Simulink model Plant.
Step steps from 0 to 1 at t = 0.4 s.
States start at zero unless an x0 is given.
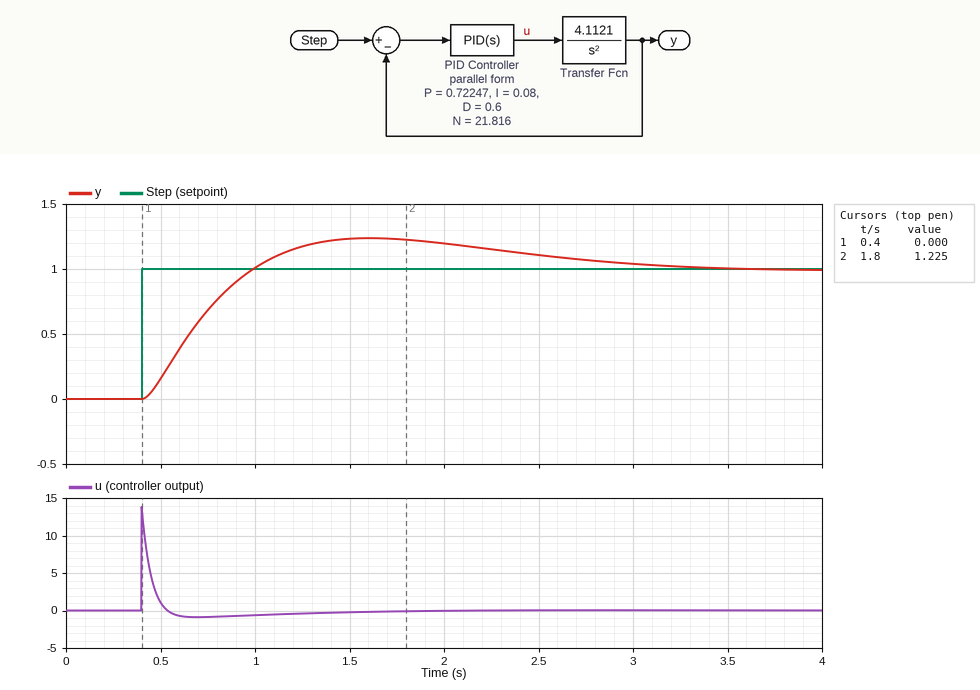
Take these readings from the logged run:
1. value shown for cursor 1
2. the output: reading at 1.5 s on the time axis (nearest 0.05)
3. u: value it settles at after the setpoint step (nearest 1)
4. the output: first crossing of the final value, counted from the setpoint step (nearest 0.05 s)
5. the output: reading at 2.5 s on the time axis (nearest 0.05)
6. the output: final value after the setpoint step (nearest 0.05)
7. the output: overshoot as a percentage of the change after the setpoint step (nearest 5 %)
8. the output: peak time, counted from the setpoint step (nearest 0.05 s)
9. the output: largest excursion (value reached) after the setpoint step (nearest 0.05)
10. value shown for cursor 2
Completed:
0.000
1.25
0
0.60 s
1.10
1.00
25 %
1.20 s
1.25
1.225
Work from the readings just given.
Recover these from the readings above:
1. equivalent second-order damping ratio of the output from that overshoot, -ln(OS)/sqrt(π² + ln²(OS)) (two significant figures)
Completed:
0.40
